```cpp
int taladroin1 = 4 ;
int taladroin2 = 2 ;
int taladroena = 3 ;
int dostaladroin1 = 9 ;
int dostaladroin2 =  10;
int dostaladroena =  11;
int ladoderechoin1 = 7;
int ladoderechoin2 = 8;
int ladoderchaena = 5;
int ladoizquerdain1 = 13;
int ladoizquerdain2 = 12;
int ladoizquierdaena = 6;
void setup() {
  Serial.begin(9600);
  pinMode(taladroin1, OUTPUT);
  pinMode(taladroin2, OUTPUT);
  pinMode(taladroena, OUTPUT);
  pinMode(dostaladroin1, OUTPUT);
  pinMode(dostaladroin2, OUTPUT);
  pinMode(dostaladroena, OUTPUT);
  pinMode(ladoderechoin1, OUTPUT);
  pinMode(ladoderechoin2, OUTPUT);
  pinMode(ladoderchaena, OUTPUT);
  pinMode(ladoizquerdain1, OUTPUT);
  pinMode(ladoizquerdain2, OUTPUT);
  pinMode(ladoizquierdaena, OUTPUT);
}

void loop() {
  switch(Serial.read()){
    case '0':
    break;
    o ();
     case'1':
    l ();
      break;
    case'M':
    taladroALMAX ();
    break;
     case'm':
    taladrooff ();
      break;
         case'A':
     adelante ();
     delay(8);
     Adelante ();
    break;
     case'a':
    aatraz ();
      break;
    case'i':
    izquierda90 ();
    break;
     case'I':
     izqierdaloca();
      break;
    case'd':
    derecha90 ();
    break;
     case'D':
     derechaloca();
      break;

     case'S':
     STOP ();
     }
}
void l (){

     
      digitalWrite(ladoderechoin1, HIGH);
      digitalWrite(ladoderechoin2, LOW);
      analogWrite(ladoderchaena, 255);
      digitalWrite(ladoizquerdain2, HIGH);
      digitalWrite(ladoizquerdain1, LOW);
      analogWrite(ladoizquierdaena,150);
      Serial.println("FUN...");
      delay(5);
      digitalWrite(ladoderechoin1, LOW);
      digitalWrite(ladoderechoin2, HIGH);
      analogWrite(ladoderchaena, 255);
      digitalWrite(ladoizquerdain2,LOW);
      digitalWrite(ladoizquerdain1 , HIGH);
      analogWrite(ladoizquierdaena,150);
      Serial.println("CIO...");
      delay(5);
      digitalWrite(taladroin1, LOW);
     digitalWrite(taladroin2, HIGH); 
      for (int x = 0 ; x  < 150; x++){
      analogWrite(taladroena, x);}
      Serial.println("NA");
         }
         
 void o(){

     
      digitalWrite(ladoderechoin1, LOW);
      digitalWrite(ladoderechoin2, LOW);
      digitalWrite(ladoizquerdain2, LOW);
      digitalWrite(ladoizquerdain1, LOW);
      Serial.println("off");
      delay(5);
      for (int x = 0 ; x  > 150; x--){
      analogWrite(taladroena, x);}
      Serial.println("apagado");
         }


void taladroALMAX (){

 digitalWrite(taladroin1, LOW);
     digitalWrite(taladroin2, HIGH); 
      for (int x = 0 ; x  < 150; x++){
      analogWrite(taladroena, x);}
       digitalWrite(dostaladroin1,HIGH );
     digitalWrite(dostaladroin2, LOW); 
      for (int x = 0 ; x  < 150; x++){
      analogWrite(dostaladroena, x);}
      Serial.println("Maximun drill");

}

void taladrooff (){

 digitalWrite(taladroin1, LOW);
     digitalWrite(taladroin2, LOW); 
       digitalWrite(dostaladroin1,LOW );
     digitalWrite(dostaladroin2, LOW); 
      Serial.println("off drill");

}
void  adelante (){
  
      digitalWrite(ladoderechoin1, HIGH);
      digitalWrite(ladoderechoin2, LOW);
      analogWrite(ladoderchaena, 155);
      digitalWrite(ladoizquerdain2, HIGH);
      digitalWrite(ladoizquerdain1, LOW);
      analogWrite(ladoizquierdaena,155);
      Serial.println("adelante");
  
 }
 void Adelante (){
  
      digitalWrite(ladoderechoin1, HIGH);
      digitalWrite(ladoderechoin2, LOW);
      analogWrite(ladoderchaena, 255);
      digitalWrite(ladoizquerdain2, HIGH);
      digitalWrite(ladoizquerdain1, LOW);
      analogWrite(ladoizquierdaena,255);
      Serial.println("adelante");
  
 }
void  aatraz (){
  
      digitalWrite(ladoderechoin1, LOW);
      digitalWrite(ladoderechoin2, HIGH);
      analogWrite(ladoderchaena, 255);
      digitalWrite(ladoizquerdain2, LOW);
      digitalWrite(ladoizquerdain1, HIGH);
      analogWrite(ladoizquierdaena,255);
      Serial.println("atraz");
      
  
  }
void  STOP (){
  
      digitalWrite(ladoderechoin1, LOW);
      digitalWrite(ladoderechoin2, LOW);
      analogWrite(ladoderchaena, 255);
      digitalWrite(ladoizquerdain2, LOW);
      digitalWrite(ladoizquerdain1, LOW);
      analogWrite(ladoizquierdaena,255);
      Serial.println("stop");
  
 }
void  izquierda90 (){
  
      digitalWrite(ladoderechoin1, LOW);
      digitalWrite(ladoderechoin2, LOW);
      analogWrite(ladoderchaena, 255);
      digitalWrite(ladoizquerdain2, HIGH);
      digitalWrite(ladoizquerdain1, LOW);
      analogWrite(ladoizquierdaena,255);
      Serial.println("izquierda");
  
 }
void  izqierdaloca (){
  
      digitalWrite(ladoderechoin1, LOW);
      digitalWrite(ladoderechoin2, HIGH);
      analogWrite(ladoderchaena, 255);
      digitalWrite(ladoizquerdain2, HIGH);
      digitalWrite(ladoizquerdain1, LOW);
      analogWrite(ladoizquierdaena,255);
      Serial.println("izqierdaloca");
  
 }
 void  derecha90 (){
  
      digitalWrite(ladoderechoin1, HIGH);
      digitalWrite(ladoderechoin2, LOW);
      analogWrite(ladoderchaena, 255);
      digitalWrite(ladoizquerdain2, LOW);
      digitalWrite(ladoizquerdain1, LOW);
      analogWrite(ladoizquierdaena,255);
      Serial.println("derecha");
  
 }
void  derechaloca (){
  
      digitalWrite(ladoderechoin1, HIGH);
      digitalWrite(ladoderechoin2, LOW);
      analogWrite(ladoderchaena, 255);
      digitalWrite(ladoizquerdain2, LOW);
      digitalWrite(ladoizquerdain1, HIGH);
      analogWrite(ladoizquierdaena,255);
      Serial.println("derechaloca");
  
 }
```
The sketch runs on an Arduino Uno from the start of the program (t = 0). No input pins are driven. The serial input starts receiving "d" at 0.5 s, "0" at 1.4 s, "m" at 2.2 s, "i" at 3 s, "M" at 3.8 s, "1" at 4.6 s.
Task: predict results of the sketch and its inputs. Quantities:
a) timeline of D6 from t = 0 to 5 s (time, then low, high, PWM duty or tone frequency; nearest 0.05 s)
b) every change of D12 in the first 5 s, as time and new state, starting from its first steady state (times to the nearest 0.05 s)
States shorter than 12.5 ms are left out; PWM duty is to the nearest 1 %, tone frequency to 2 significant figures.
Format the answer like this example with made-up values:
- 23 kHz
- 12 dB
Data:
- 0 s low; 0.5 s high; 4.6 s PWM 59 %
- 0 s low; 3 s high; 4.6 s low
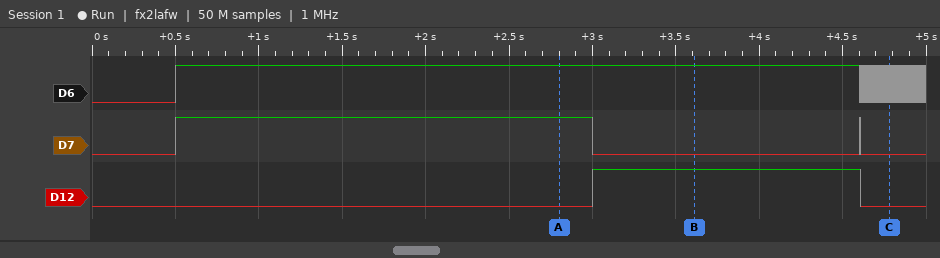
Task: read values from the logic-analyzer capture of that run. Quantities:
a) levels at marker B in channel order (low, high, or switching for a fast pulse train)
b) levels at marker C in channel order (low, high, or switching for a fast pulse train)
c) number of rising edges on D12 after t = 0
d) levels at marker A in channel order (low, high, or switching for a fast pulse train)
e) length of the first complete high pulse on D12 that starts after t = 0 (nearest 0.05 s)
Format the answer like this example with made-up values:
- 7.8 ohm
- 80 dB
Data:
- D6 high, D7 low, D12 high
- D6 switching, D7 low, D12 low
- 1
- D6 high, D7 high, D12 low
- 1.60 s
